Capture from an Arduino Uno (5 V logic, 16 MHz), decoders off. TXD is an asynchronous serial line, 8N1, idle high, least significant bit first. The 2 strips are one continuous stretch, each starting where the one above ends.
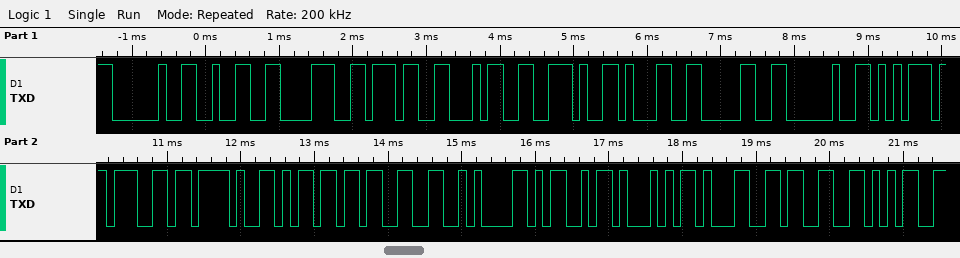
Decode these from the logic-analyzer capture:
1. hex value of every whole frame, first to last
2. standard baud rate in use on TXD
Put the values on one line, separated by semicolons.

20 32 38 37 34 2E 31 30 20 75 67 2F 6D 33 0A 4D 51 31 33 35; 9600 baud
